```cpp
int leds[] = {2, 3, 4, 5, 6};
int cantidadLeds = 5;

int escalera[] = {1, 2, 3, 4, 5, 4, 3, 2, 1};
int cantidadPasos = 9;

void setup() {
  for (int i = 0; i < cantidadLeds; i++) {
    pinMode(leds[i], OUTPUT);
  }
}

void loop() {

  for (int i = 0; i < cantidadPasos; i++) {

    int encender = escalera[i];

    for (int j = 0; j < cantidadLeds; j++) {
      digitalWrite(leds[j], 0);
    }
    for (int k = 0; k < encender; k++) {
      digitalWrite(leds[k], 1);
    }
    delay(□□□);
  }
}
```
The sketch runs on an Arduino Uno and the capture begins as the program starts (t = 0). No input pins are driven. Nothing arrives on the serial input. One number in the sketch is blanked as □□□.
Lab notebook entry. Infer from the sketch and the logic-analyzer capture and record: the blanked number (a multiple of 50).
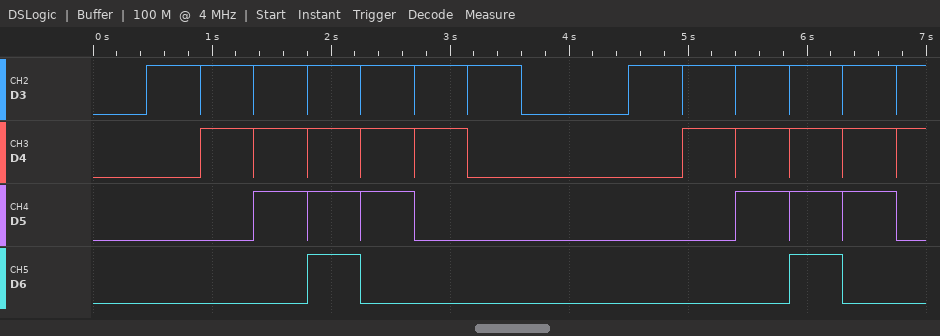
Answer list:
450
